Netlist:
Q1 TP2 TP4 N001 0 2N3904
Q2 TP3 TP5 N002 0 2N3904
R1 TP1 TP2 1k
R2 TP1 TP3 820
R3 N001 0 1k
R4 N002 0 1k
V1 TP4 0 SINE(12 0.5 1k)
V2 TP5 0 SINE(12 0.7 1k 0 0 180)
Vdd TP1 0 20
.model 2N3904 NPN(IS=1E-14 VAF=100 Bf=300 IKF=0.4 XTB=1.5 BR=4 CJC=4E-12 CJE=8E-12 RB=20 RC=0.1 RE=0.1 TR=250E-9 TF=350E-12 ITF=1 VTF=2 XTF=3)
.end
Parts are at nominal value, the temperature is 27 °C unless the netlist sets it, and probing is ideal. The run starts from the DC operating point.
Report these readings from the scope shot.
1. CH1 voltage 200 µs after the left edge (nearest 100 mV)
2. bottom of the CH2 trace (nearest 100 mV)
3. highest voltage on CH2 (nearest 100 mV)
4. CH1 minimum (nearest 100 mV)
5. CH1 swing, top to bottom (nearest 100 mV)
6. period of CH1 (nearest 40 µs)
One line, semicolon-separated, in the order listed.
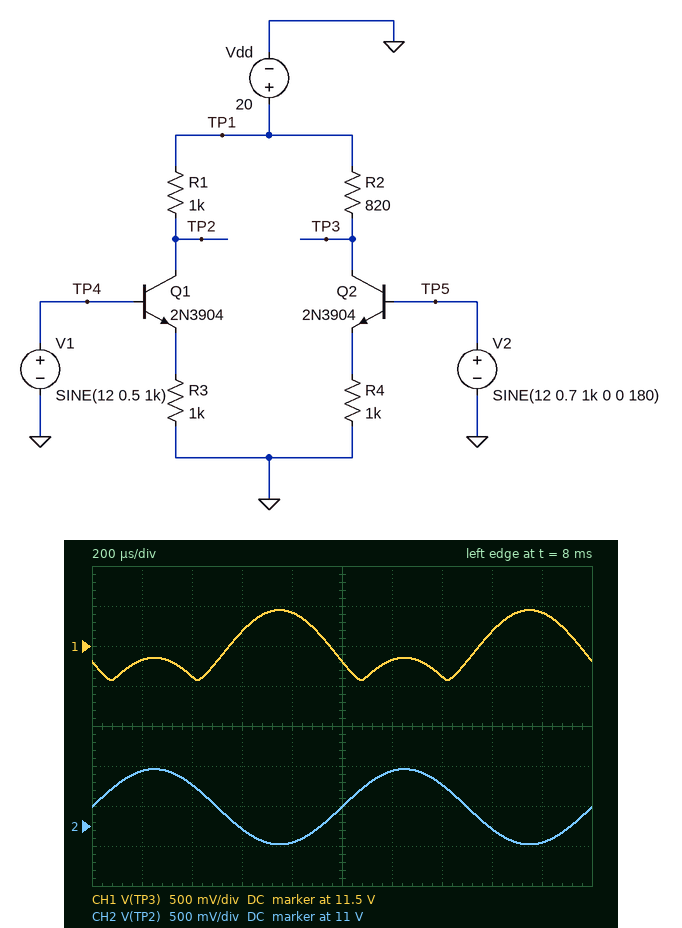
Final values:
11.3 V; 10.8 V; 11.7 V; 11.1 V; 900 mV; 1.00 ms
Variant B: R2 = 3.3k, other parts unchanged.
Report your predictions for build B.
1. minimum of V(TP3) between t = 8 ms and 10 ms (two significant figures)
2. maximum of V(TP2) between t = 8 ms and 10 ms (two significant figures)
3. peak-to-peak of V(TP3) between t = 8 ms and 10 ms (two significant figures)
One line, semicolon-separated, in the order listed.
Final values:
10 V; 12 V; 1.4 V
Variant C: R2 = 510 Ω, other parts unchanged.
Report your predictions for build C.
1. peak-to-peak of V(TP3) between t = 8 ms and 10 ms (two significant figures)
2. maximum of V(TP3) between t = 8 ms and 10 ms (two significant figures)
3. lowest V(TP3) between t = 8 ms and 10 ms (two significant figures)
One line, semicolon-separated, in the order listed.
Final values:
710 mV; 15 V; 14 V
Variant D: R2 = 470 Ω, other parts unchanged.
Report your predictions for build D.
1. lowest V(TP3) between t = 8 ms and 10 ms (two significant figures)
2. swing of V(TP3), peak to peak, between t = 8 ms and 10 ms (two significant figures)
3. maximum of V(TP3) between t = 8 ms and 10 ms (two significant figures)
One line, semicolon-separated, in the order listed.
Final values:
14 V; 650 mV; 15 V
